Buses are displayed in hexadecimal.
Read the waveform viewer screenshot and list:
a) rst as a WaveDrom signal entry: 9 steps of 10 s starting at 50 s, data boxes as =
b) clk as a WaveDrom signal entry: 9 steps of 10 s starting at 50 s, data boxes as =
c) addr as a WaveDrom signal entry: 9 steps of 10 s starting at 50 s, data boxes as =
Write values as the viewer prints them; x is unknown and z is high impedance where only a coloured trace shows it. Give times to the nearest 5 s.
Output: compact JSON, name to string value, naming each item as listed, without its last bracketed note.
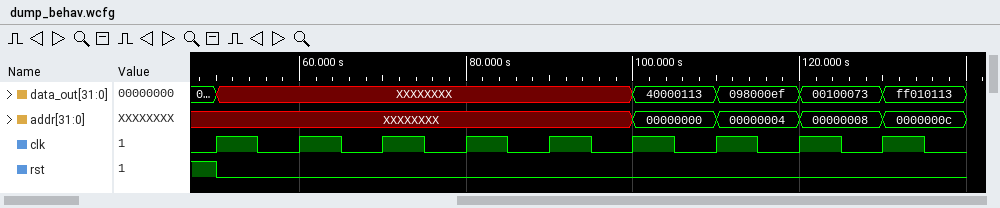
{"rst as a WaveDrom signal entry: 9 steps of 10 s starting at 50 s, data boxes as =": "{name: 'rst', wave: '0........'}", "clk as a WaveDrom signal entry: 9 steps of 10 s starting at 50 s, data boxes as =": "{name: 'clk', wave: 'p........'}", "addr as a WaveDrom signal entry: 9 steps of 10 s starting at 50 s, data boxes as =": "{name: 'addr', wave: 'x....====', data: '00000000 00000004 00000008 0000000c'}"}
